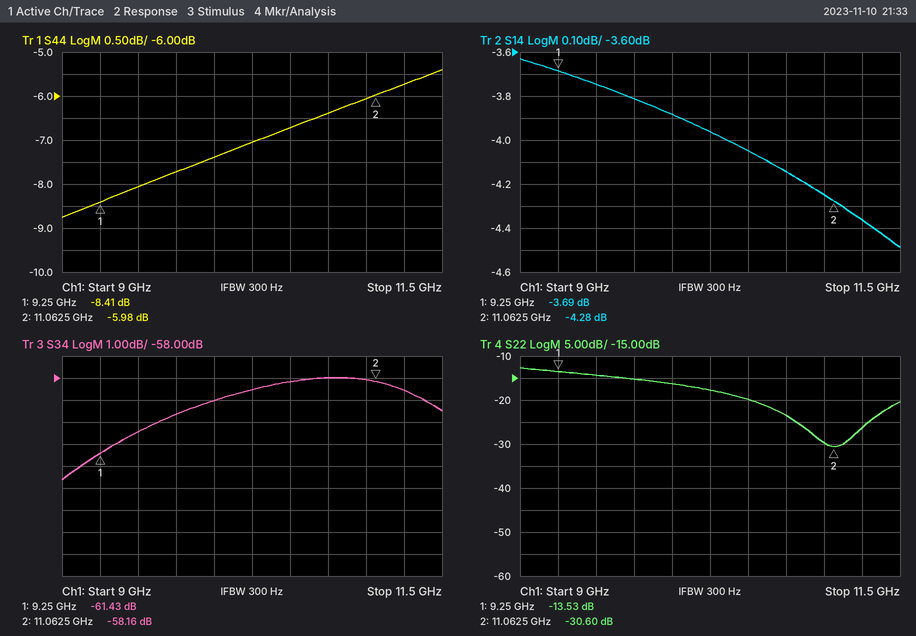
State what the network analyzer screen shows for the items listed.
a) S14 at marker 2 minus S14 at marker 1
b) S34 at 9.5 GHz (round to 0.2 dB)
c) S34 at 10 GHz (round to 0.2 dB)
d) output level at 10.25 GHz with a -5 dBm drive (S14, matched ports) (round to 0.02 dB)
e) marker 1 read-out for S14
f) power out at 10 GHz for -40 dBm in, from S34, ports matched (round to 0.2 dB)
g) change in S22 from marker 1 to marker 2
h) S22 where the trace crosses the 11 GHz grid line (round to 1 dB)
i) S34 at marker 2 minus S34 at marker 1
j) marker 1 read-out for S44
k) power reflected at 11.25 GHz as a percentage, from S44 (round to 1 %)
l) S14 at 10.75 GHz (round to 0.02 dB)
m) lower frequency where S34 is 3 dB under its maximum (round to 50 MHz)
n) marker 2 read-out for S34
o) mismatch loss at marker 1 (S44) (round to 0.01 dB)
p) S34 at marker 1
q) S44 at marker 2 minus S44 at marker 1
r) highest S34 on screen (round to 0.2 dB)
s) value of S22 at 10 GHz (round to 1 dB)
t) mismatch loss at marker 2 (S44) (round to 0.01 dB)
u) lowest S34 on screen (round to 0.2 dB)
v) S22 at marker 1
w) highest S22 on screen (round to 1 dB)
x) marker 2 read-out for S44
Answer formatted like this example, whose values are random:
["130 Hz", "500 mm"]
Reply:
["-0.59 dB", "-60.4 dB", "-59.0 dB", "-8.96 dBm", "-3.69 dB", "-99.0 dBm", "-17.07 dB", "-30 dB", "3.27 dB", "-8.41 dB", "27 %", "-4.14 dB", "9.35 GHz", "-58.16 dB", "0.68 dB", "-61.43 dB", "2.43 dB", "-58.0 dB", "-16 dB", "1.26 dB", "-62.6 dB", "-13.53 dB", "-13 dB", "-5.98 dB"]
